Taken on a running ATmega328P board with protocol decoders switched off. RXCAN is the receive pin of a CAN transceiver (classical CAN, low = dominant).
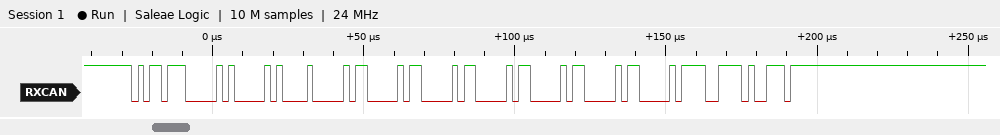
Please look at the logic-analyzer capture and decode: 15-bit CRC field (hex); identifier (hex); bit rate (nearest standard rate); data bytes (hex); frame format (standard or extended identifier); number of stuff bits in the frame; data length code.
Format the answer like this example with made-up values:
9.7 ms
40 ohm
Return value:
0x73D3
0x5B8
500 kbit/s
10 81 81 81 81 81 81 81
standard
9
8
